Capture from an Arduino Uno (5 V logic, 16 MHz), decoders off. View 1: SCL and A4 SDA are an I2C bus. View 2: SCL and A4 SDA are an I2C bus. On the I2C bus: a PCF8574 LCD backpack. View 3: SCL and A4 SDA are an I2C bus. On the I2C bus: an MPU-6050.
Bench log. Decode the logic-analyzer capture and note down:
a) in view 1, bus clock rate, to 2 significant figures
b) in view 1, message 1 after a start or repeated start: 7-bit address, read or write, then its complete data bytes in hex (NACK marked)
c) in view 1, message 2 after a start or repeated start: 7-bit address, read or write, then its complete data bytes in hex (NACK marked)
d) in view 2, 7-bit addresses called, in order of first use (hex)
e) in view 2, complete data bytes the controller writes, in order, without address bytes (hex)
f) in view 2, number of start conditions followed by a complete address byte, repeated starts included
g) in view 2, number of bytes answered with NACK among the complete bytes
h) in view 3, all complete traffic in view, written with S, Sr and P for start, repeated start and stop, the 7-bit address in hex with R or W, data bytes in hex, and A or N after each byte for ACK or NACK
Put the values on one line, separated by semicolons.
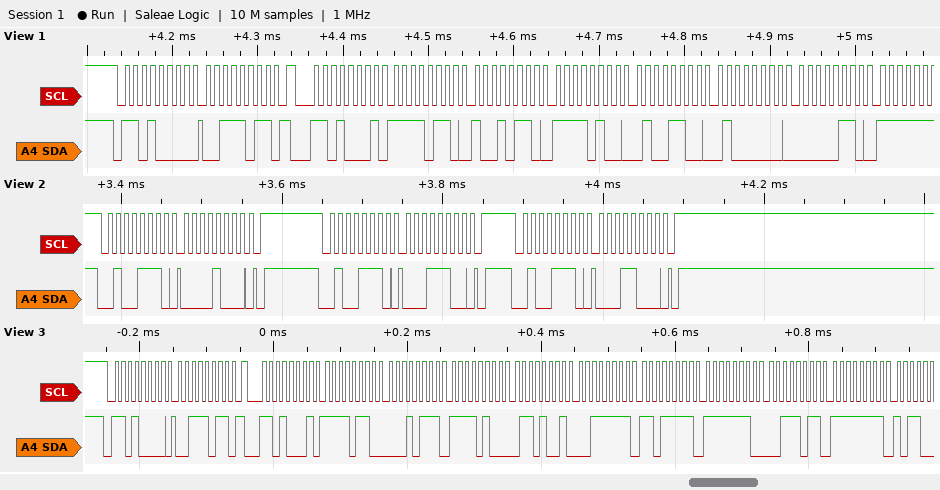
100 kHz; 0x68 write: 3B; 0x68 read: F6 96 F4 4C 40 06; 0x27; 08 1C 18; 3; 0; S 68W A 3B A Sr 68R A F6 A 17 A F4 A 69 A 3F A DF A FE A 3B A FF A
